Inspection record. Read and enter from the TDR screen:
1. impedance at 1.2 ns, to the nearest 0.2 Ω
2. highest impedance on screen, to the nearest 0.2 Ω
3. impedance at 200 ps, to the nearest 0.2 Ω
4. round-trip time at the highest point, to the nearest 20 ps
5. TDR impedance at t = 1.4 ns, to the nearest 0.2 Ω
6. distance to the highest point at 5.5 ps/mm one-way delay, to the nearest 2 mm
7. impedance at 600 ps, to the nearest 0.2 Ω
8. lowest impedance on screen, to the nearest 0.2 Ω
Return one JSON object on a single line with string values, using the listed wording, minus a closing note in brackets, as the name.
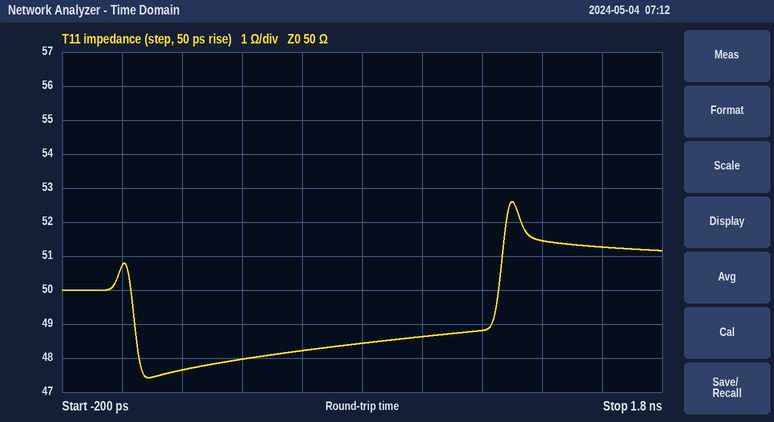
{"impedance at 1.2 ns, to the nearest 0.2 Ω": "48.8 Ω", "highest impedance on screen, to the nearest 0.2 Ω": "52.6 Ω", "impedance at 200 ps, to the nearest 0.2 Ω": "47.6 Ω", "round-trip time at the highest point, to the nearest 20 ps": "1.30 ns", "TDR impedance at t = 1.4 ns, to the nearest 0.2 Ω": "51.4 Ω", "distance to the highest point at 5.5 ps/mm one-way delay, to the nearest 2 mm": "118 mm", "impedance at 600 ps, to the nearest 0.2 Ω": "48.2 Ω", "lowest impedance on screen, to the nearest 0.2 Ω": "47.4 Ω"}
